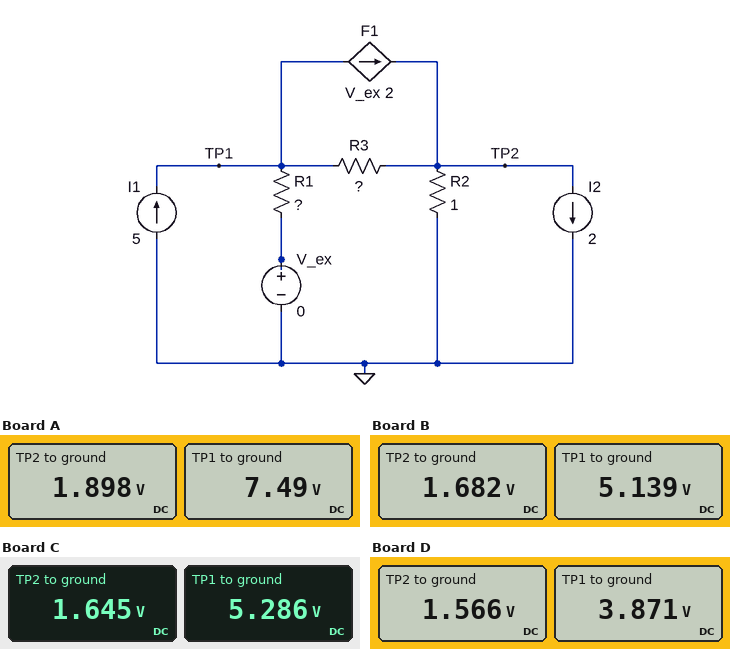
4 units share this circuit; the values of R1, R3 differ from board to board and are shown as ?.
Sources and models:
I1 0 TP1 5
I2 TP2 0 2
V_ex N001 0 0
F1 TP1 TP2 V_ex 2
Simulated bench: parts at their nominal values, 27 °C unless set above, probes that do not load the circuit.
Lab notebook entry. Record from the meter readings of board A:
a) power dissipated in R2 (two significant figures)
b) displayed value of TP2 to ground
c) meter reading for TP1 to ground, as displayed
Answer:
3.6 W
1.898 V
7.49 V
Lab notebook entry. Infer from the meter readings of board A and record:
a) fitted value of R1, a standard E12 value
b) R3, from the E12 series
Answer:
6.8 Ω
3.3 Ω
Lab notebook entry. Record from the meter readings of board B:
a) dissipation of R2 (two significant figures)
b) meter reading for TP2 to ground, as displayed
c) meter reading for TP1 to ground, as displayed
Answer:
2.8 W
1.682 V
5.139 V
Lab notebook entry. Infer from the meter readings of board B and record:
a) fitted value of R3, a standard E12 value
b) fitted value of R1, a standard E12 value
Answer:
3.3 Ω
3.9 Ω
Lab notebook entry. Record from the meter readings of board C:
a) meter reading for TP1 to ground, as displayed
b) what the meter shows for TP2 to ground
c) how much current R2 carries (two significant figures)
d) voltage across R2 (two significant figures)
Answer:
5.286 V
1.645 V
1.6 A
1.6 V
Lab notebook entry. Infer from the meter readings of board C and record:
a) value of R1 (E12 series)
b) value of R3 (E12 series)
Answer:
3.9 Ω
3.9 Ω
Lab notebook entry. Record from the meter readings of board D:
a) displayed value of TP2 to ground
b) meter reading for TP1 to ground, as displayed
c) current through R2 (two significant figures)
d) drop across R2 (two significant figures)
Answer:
1.566 V
3.871 V
1.6 A
1.6 V
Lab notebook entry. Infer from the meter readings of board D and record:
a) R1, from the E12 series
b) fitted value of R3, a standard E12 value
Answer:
2.7 Ω
3.3 Ω
